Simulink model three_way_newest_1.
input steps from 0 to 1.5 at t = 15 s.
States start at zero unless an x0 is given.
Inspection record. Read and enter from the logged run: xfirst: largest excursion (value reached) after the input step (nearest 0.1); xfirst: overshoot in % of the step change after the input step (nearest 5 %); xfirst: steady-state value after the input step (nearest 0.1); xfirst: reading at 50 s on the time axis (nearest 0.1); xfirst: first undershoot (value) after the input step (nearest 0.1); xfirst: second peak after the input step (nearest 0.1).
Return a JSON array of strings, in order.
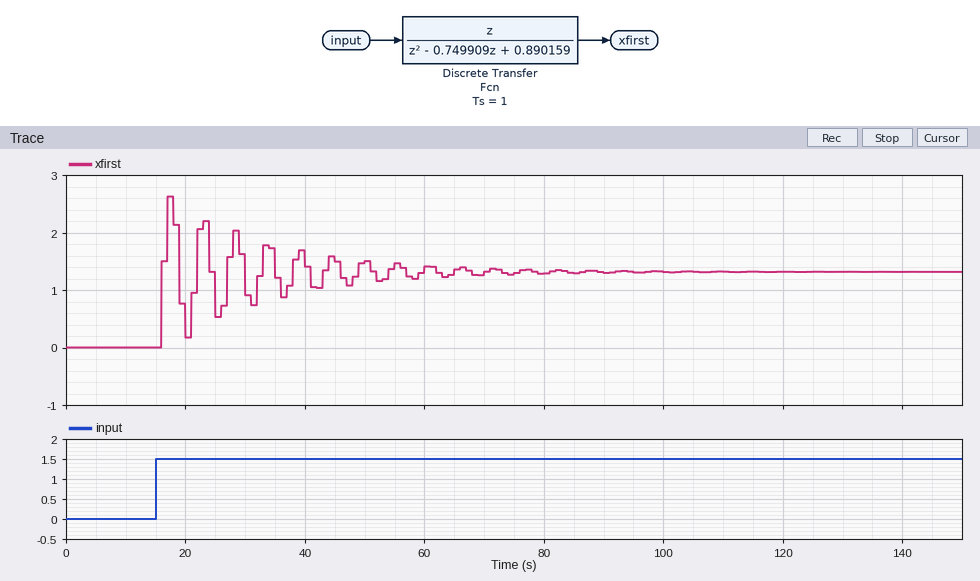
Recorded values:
["2.6", "100 %", "1.3", "1.5", "0.2", "2.2"]
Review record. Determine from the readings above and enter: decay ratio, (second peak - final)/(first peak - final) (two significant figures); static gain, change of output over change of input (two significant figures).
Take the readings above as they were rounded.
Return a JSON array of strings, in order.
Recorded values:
["0.69", "0.87"]
